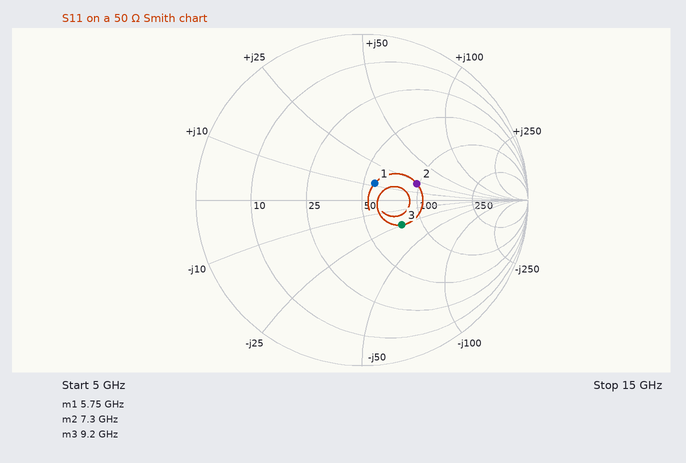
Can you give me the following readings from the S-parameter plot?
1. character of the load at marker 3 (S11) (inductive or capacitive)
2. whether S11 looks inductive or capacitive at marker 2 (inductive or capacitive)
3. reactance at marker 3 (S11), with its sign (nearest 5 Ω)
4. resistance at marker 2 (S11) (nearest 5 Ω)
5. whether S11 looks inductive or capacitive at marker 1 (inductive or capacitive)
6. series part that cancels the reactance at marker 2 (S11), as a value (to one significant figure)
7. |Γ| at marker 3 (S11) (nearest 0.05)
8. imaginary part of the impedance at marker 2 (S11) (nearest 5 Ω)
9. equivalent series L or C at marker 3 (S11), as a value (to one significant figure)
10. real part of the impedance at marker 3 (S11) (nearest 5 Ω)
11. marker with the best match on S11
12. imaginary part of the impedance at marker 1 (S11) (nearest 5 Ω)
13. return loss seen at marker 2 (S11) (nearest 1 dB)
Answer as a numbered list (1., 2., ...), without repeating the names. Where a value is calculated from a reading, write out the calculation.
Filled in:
1. capacitive
2. inductive
3. -25 Ω
4. 95 Ω
5. inductive
6. C = 1/(2π × 7.3 GHz × 20 Ω) ≈ 1 pF
7. 0.30
8. +20 Ω
9. C = 1/(2π × 9.2 GHz × 25 Ω) ≈ 692 fF, so 700 fF to one significant figure
10. 75 Ω
11. marker 1
12. +10 Ω
13. 9 dB
